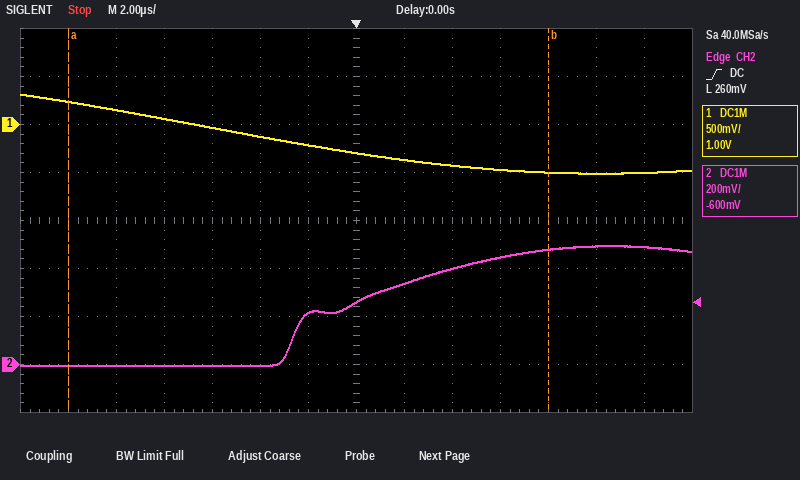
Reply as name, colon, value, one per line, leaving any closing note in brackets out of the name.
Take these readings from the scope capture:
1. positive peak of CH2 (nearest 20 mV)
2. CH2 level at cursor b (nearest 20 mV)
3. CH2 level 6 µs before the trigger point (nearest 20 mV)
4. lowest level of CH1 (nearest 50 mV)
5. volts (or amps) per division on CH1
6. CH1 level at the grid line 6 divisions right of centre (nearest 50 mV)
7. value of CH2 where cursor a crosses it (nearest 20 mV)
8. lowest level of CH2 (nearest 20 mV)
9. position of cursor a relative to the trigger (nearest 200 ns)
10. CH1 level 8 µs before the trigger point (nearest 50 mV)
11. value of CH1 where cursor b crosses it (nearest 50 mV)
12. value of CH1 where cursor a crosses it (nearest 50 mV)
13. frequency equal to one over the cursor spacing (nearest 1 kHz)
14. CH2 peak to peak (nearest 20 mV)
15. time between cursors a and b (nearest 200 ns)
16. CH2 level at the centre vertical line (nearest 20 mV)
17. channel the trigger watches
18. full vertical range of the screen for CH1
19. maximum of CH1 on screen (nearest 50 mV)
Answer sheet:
positive peak of CH2: 500 mV
CH2 level at cursor b: 480 mV
CH2 level 6 µs before the trigger point: 0 mV
lowest level of CH1: -500 mV
volts (or amps) per division on CH1: 500 mV
CH1 level at the grid line 6 divisions right of centre: -500 mV
value of CH2 where cursor a crosses it: 0 mV
lowest level of CH2: 0 mV
position of cursor a relative to the trigger: -12.0 µs
CH1 level 8 µs before the trigger point: 50 mV
value of CH1 where cursor b crosses it: -500 mV
value of CH1 where cursor a crosses it: 250 mV
frequency equal to one over the cursor spacing: 50 kHz
CH2 peak to peak: 500 mV
time between cursors a and b: 20.0 µs
CH2 level at the centre vertical line: 260 mV
channel the trigger watches: CH2
full vertical range of the screen for CH1: 4 V
maximum of CH1 on screen: 300 mV
